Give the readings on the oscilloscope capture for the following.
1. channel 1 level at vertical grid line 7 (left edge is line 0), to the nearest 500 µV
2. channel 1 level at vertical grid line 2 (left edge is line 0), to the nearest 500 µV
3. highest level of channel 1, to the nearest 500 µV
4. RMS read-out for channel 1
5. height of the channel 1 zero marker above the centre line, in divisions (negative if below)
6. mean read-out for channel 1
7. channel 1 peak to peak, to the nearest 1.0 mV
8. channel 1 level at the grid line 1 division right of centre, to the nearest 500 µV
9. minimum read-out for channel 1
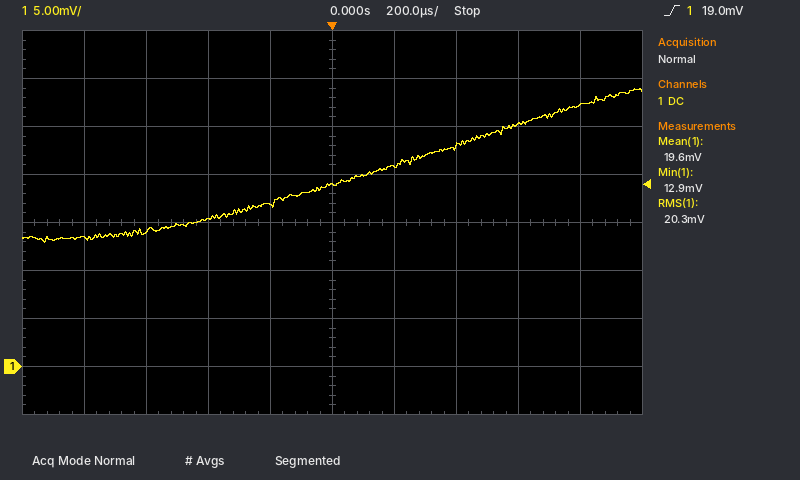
23.0 mV
14.0 mV
29.0 mV
20.3 mV
-3.0 div
19.6 mV
16.0 mV
21.0 mV
12.9 mV
